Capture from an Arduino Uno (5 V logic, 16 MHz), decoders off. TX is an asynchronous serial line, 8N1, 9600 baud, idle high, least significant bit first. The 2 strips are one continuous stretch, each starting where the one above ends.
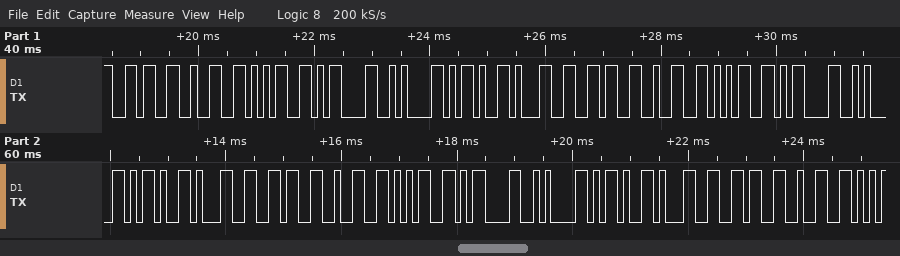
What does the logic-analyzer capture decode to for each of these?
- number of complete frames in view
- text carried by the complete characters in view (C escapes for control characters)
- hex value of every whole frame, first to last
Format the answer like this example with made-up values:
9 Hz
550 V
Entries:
23
"625\r\n-1625\r\n-1625\r\n-162"
36 32 35 0D 0A 2D 31 36 32 35 0D 0A 2D 31 36 32 35 0D 0A 2D 31 36 32
